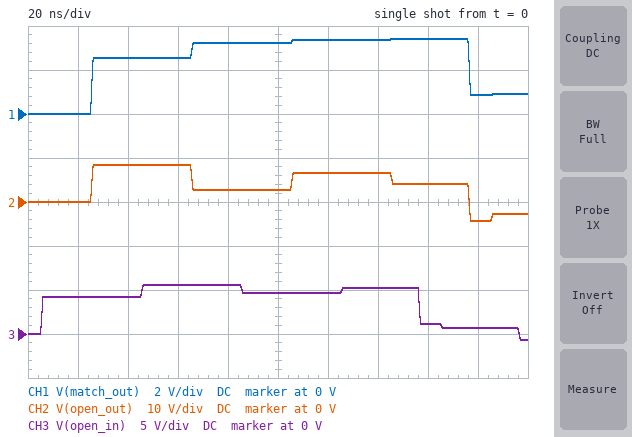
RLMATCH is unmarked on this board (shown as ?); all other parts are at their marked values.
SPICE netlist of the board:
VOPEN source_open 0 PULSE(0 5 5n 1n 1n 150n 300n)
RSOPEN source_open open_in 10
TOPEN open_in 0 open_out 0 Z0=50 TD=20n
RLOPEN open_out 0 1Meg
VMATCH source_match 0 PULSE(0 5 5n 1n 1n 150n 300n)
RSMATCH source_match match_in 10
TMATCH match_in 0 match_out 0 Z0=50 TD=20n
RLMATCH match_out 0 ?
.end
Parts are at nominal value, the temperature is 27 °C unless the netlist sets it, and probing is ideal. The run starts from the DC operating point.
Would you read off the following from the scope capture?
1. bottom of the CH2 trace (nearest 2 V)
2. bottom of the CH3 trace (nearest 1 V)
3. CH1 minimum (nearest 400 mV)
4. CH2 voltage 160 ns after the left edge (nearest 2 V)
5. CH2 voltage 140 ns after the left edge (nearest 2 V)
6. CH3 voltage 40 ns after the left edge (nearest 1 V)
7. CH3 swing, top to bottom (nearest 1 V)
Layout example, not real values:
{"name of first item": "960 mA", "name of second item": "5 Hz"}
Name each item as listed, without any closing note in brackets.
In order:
{"bottom of the CH2 trace": "-4 V", "bottom of the CH3 trace": "-1 V", "CH1 minimum": "0 V", "CH2 voltage 160 ns after the left edge": "4 V", "CH2 voltage 140 ns after the left edge": "6 V", "CH3 voltage 40 ns after the left edge": "4 V", "CH3 swing, top to bottom": "6 V"}
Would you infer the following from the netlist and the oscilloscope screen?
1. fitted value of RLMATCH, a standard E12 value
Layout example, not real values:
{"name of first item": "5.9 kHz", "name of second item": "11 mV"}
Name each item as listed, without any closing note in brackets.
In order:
{"fitted value of RLMATCH, a standard E12 value": "22 Ω"}
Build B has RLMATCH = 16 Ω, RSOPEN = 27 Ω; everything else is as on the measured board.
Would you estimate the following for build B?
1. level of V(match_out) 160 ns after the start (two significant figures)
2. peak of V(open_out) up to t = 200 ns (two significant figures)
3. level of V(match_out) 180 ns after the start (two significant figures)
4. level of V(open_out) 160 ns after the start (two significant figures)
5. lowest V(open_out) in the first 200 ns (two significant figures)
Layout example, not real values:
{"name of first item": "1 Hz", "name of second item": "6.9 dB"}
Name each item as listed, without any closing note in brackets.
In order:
{"level of V(match_out) 160 ns after the start": "3.0 V", "peak of V(open_out) up to t = 200 ns": "6.5 V", "level of V(match_out) 180 ns after the start": "1.0 V", "level of V(open_out) 160 ns after the start": "5.0 V", "lowest V(open_out) in the first 200 ns": "-1.5 V"}
